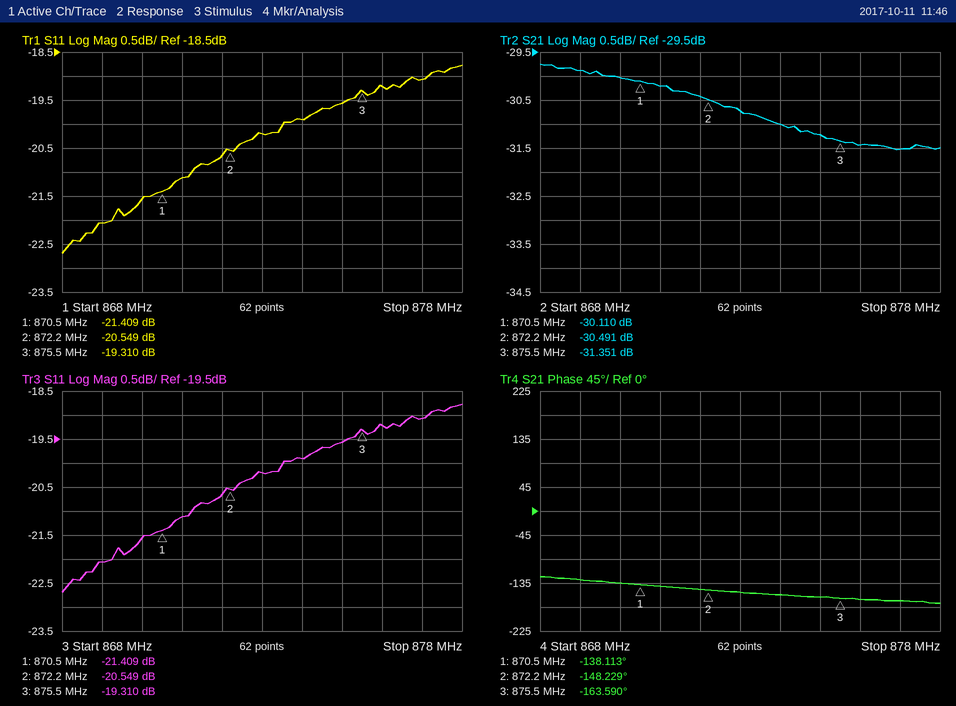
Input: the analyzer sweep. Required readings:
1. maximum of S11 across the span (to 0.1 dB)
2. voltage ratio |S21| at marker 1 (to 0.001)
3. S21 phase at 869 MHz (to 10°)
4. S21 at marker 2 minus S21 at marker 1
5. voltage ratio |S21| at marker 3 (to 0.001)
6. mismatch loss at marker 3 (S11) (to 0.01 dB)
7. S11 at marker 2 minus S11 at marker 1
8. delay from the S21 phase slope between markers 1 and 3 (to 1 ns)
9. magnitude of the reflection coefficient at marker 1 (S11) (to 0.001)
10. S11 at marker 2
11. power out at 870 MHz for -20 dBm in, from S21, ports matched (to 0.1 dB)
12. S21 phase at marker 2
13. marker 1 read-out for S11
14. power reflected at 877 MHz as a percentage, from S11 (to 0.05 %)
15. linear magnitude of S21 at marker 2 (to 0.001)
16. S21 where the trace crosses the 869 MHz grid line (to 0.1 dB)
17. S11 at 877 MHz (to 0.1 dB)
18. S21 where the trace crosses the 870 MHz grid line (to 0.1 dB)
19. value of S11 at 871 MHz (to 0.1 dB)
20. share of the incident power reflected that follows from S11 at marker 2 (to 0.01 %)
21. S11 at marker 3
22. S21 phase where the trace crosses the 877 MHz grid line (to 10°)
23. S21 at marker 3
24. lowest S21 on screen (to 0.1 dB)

-18.8 dB
0.031
-130°
-0.381 dB
0.027
0.05 dB
0.860 dB
14 ns
0.085
-20.549 dB
-50.0 dBm
-148.229°
-21.409 dB
1.25 %
0.030
-29.9 dB
-19.1 dB
-30.0 dB
-21.1 dB
0.88 %
-19.310 dB
-170°
-31.351 dB
-31.5 dB
